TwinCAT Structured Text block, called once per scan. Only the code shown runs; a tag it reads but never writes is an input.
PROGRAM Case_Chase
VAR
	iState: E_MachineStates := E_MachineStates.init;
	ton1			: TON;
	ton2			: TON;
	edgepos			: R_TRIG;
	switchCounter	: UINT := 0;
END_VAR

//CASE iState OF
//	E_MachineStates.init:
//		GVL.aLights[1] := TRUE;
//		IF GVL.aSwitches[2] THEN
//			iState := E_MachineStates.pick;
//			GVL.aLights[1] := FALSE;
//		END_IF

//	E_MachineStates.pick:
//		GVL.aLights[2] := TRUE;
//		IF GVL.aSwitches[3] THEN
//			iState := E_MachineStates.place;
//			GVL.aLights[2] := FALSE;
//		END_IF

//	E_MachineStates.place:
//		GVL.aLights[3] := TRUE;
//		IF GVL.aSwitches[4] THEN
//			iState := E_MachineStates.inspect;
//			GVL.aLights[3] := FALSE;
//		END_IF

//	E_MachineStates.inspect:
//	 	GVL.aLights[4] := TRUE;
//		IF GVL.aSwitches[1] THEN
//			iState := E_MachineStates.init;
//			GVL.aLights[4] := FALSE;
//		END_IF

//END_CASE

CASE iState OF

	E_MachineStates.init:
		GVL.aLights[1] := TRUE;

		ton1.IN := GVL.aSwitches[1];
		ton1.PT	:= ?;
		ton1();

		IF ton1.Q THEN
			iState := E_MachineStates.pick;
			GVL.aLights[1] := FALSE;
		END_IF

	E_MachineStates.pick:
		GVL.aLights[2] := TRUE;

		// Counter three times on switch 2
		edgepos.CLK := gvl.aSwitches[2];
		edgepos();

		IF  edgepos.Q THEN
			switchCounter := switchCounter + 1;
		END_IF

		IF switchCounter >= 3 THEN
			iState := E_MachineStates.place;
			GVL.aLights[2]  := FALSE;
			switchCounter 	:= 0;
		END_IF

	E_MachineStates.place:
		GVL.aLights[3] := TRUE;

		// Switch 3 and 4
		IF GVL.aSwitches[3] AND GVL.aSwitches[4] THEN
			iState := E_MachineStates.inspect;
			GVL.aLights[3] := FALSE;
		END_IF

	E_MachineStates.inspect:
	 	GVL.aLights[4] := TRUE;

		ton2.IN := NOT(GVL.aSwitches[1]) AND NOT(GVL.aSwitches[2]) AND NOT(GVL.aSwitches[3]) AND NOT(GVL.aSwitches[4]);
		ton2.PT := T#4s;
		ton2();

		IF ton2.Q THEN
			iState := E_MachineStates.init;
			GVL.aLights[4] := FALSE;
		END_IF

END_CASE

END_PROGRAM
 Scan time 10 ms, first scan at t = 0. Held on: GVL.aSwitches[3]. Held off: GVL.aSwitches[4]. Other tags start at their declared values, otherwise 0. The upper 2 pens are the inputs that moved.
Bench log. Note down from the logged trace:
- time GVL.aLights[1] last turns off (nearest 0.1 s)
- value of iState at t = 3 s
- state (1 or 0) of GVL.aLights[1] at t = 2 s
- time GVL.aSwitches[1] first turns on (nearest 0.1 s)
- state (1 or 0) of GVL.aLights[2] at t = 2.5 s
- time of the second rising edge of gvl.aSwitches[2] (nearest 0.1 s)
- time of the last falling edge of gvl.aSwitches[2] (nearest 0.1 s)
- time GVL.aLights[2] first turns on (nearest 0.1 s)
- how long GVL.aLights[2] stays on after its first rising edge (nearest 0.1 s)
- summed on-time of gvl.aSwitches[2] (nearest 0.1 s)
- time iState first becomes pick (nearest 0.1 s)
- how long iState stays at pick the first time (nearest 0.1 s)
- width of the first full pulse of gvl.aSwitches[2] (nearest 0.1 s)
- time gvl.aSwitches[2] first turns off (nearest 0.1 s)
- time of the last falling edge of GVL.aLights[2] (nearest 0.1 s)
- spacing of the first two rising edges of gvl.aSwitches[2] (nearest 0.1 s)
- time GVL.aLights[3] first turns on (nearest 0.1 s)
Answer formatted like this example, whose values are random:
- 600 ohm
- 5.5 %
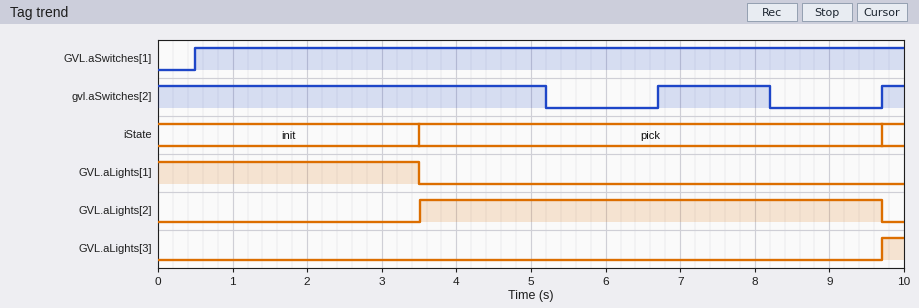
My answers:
- 3.5 s
- init
- 1
- 0.5 s
- 0
- 9.7 s
- 8.2 s
- 3.5 s
- 6.2 s
- 7.0 s
- 3.5 s
- 6.2 s
- 1.5 s
- 5.2 s
- 9.7 s
- 3.0 s
- 9.7 s
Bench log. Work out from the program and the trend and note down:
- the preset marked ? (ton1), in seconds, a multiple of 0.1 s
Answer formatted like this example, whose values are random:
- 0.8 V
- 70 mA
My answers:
- 3.0 s
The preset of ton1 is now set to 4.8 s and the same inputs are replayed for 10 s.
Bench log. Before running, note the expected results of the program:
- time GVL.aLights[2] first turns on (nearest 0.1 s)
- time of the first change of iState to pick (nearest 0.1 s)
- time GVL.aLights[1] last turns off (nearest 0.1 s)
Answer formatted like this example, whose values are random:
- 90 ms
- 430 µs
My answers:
- 5.3 s
- 5.3 s
- 5.3 s
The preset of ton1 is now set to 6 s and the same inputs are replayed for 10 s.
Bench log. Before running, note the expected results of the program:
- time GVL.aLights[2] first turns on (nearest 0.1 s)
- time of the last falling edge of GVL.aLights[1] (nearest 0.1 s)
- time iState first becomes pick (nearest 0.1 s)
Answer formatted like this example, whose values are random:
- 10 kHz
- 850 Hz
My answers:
- 6.5 s
- 6.5 s
- 6.5 s
